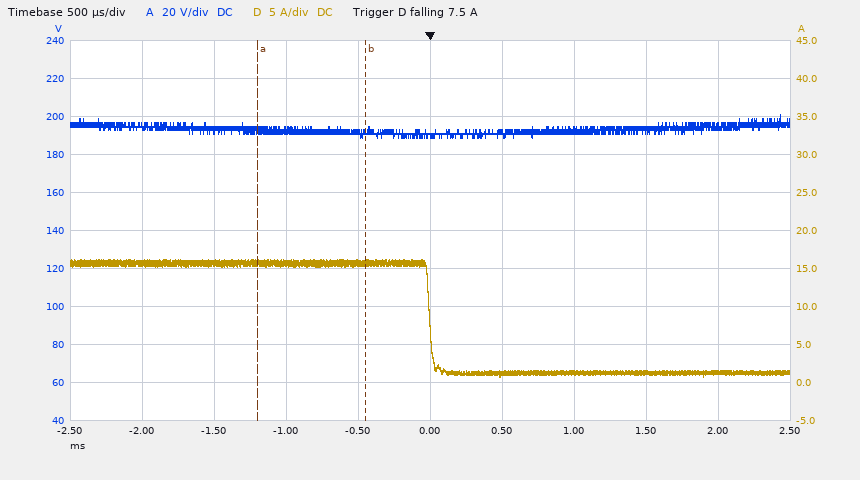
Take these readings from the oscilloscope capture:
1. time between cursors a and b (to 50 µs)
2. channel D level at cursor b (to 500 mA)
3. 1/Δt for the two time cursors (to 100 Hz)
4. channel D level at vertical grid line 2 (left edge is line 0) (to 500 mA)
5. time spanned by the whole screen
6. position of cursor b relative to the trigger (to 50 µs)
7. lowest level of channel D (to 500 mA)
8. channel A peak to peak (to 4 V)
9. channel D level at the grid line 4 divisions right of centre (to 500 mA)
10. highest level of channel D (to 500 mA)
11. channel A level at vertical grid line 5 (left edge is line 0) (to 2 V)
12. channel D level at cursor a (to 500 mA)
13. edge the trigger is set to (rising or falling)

750 µs
16.0 A
1.3 kHz
16.0 A
5 ms
-450 µs
1.0 A
12 V
1.5 A
16.0 A
190 V
16.0 A
falling
